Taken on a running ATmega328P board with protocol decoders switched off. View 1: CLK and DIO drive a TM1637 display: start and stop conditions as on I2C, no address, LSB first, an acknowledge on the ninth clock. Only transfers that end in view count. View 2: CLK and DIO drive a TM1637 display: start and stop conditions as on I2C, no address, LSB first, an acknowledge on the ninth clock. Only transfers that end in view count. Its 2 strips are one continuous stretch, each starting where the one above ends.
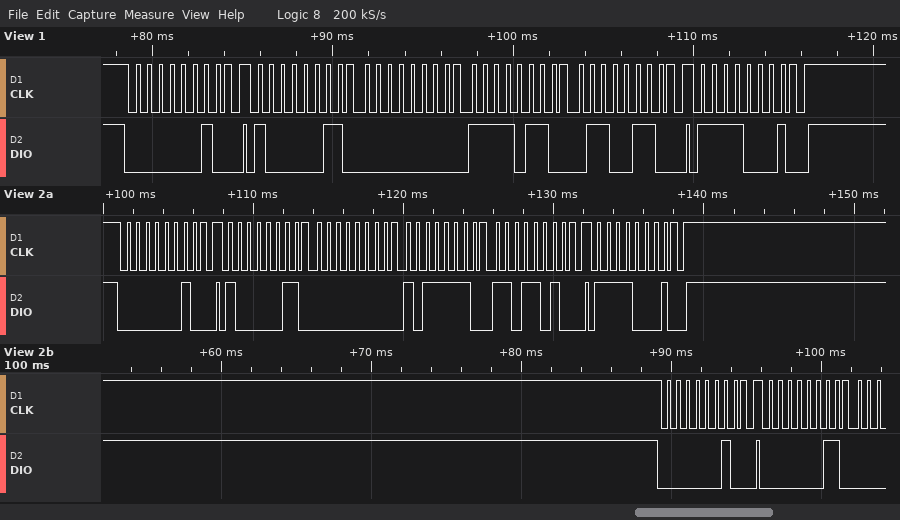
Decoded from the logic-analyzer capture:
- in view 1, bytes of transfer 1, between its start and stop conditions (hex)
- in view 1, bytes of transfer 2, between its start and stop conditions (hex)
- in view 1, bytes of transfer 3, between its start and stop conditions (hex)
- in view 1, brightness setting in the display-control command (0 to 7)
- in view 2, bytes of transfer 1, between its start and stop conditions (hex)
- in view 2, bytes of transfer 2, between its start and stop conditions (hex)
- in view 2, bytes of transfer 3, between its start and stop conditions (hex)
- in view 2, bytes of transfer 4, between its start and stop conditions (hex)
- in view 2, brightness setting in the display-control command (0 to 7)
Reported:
40
C1 00 6F 66
8F
7
40
C1 00 7D 5B
8F
40
7
